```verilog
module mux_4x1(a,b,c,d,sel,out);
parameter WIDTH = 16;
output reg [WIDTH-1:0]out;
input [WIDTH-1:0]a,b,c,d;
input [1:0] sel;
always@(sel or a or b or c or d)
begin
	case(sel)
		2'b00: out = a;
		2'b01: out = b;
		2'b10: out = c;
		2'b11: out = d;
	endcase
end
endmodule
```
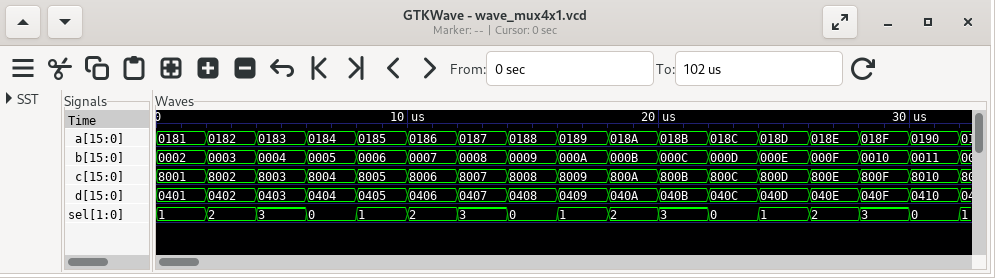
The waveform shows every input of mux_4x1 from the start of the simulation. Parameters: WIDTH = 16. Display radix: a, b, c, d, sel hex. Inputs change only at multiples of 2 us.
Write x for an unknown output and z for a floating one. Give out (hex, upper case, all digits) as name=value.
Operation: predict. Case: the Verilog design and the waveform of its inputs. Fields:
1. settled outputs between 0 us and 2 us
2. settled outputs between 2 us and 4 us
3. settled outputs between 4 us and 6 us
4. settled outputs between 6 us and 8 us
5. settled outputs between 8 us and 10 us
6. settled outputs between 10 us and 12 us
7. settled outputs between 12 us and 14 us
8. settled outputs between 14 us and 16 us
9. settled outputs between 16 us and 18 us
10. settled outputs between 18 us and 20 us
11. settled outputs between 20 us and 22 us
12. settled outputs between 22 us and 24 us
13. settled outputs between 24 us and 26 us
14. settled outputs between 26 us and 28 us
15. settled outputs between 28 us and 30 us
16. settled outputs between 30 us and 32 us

out=0002
out=8002
out=0403
out=0184
out=0006
out=8006
out=0407
out=0188
out=000A
out=800A
out=040B
out=018C
out=000E
out=800E
out=040F
out=0190
